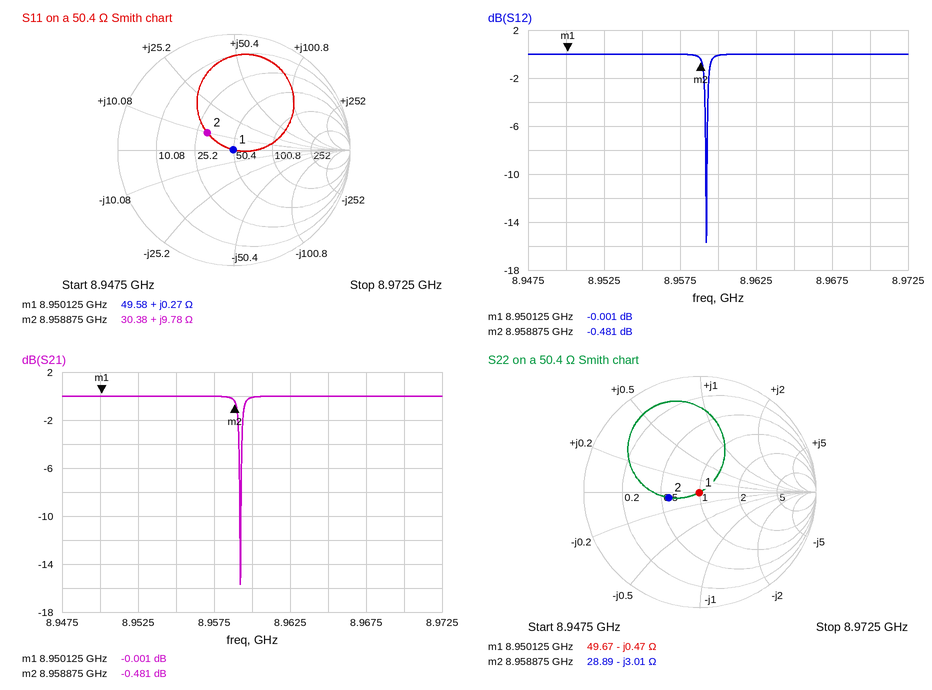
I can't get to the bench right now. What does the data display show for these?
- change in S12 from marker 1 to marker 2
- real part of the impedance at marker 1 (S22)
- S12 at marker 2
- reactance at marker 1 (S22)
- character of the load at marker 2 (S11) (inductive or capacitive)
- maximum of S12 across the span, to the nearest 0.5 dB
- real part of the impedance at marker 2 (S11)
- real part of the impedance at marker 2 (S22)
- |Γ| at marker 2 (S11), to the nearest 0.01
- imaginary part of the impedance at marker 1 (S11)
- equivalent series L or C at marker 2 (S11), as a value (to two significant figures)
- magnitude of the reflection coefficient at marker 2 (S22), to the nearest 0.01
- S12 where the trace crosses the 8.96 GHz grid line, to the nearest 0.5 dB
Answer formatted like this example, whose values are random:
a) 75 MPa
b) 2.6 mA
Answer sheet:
a) -0.480 dB
b) 49.67 Ω
c) -0.481 dB
d) -0.47 Ω
e) inductive
f) 0.0 dB
g) 30.38 Ω
h) 28.89 Ω
i) 0.27
j) +0.27 Ω
k) 170 pH
l) 0.27
m) 0.0 dB
